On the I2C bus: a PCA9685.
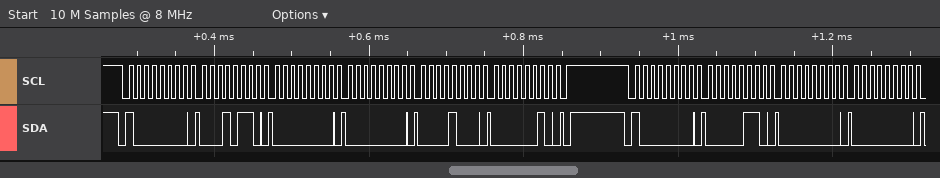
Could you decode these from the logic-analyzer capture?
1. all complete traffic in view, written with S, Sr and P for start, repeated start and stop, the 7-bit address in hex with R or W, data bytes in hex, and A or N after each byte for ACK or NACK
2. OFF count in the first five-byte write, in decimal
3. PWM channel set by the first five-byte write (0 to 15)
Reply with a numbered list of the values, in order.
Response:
1. S 40W A 16 A 00 A 00 A 08 A 02 A P S 40W A 06 A 00 A 00 A
2. 520
3. 4
